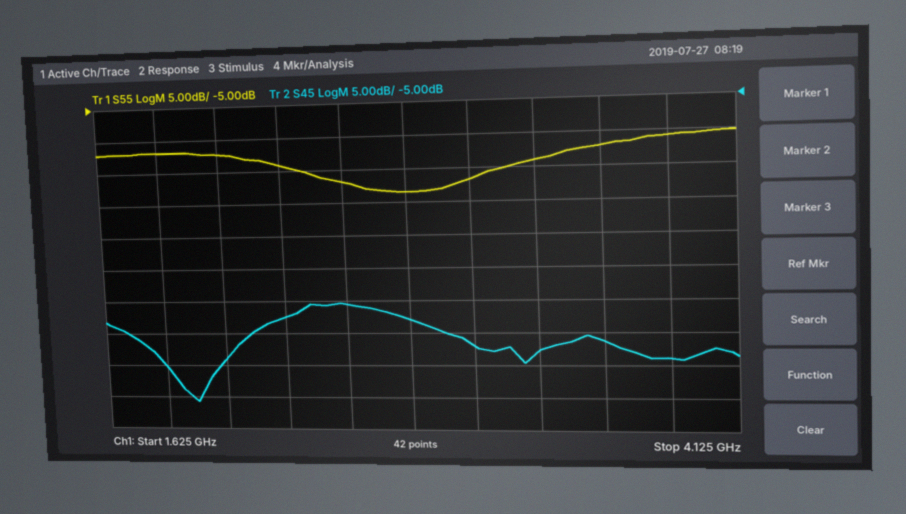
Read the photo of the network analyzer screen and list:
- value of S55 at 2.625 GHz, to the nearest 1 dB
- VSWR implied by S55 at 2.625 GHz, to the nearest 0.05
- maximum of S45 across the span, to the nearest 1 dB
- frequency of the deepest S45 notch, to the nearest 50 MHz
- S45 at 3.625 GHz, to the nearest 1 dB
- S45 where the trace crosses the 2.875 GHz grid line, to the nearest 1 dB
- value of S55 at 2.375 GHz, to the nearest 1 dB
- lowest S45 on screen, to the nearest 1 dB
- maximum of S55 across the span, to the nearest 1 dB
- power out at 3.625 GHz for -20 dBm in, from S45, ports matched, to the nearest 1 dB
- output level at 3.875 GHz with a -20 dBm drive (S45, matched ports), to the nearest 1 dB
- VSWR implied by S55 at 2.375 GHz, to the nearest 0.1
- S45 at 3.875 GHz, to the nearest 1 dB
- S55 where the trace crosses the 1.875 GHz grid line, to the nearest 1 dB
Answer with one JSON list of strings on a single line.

["-17 dB", "1.35", "-35 dB", "2.00 GHz", "-41 dB", "-38 dB", "-14 dB", "-51 dB", "-10 dB", "-61 dBm", "-64 dBm", "1.5", "-44 dB", "-12 dB"]
